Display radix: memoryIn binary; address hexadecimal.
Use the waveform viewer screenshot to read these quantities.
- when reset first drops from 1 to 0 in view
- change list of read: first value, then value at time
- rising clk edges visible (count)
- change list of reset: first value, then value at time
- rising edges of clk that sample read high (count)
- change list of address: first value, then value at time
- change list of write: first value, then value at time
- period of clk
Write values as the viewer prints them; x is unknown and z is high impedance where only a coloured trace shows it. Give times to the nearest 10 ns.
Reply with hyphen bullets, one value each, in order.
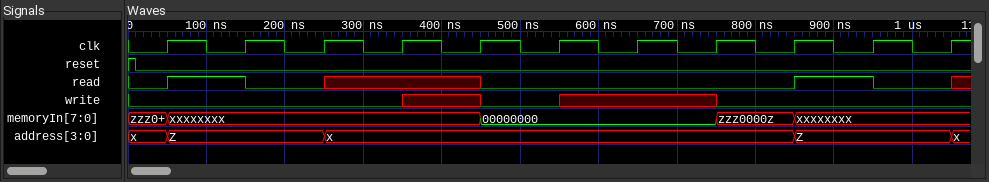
- 10 ns
- 0, 1 at 50 ns, 0 at 150 ns, x at 250 ns, 0 at 450 ns, 1 at 850 ns, 0 at 950 ns, x at 1050 ns
- 11
- 1, 0 at 10 ns
- 2
- x, Z at 50 ns, x at 250 ns, Z at 850 ns, x at 1050 ns
- 0, x at 350 ns, 0 at 450 ns, x at 550 ns, 0 at 750 ns
- 100 ns
